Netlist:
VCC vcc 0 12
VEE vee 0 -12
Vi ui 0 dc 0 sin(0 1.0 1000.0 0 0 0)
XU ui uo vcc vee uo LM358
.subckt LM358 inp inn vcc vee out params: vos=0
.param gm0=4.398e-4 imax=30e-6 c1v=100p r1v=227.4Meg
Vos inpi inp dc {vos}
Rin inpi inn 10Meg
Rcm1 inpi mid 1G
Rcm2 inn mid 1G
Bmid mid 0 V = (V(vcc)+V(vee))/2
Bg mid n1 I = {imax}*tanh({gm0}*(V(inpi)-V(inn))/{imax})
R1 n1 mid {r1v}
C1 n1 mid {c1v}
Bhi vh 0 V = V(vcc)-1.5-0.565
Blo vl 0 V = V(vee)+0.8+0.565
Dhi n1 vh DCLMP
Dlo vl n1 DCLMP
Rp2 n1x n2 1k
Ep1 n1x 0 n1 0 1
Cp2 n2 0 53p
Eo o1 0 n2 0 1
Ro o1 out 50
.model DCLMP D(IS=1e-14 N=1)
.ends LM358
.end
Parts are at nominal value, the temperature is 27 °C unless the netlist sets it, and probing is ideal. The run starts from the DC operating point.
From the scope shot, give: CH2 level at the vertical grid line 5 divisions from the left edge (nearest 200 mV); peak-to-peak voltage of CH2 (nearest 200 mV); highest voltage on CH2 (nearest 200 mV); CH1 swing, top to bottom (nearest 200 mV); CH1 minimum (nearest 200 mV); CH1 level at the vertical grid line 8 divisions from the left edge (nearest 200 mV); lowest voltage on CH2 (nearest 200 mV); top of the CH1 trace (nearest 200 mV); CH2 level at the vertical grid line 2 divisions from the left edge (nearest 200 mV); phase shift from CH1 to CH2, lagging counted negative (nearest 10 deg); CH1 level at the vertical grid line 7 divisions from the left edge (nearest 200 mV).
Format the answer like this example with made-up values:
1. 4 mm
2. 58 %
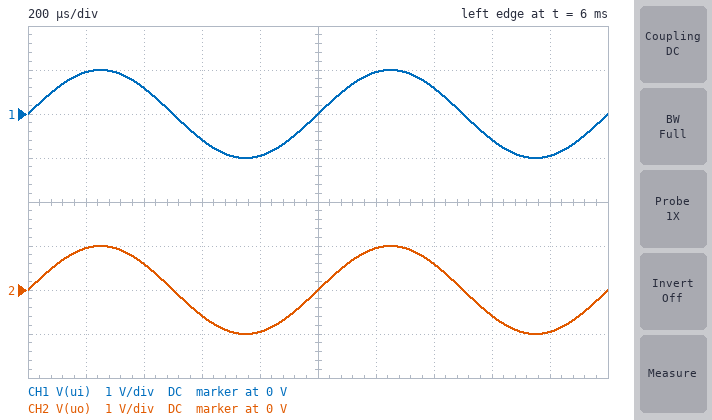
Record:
1. 0 V
2. 2.0 V
3. 1.0 V
4. 2.0 V
5. -1.0 V
6. -600 mV
7. -1.0 V
8. 1.0 V
9. 600 mV
10. 0 deg
11. 600 mV
